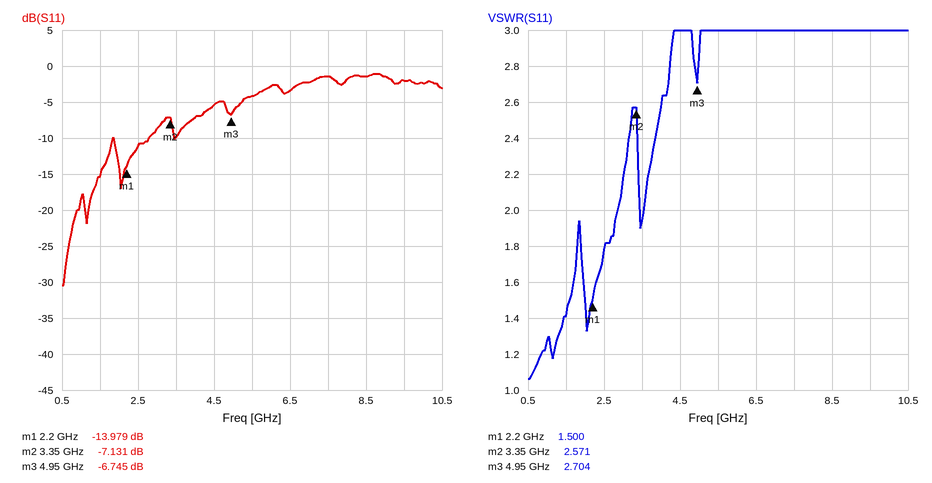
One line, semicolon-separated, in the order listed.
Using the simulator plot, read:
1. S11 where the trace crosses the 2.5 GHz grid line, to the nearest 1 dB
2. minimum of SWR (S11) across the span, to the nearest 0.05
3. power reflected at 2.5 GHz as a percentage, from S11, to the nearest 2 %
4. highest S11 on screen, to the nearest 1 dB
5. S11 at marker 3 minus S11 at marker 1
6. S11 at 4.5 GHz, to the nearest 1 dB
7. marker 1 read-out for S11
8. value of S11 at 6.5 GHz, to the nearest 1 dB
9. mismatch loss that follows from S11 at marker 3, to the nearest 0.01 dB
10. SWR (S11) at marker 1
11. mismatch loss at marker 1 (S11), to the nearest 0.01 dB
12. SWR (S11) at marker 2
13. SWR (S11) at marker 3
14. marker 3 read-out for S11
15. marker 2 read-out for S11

-11 dB; 1.05; 8 %; -1 dB; 7.234 dB; -5 dB; -13.979 dB; -3 dB; 1.03 dB; 1.500; 0.18 dB; 2.571; 2.704; -6.745 dB; -7.131 dB
